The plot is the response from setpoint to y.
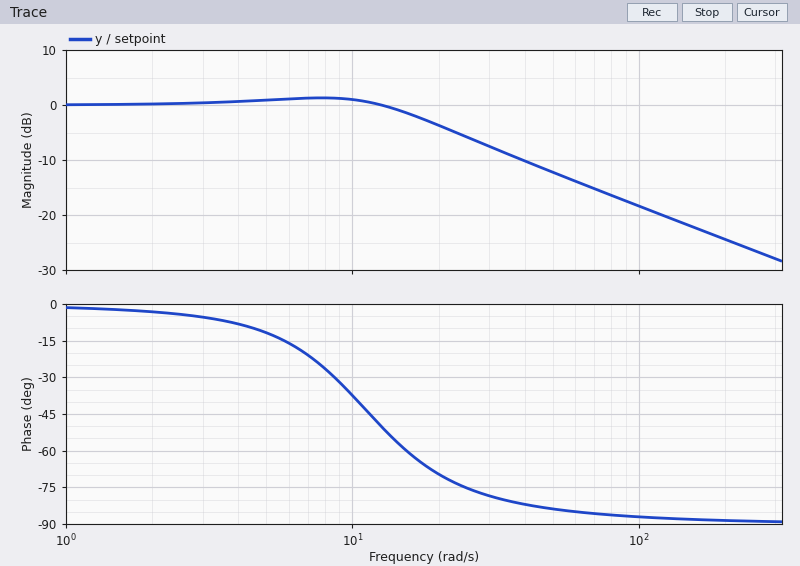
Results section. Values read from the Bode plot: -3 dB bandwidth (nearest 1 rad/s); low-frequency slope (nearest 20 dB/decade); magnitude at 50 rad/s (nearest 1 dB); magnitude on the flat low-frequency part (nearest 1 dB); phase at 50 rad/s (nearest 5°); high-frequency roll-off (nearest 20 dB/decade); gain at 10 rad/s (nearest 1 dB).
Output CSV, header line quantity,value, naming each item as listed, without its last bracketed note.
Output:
quantity,value
-3 dB bandwidth,18 rad/s
low-frequency slope,0 dB/decade
magnitude at 50 rad/s,-12 dB
magnitude on the flat low-frequency part,0 dB
phase at 50 rad/s,-85°
high-frequency roll-off,-20 dB/decade
gain at 10 rad/s,1 dB
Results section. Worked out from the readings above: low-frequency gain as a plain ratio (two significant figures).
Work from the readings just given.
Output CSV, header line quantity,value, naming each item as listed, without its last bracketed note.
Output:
quantity,value
low-frequency gain as a plain ratio,1.0
